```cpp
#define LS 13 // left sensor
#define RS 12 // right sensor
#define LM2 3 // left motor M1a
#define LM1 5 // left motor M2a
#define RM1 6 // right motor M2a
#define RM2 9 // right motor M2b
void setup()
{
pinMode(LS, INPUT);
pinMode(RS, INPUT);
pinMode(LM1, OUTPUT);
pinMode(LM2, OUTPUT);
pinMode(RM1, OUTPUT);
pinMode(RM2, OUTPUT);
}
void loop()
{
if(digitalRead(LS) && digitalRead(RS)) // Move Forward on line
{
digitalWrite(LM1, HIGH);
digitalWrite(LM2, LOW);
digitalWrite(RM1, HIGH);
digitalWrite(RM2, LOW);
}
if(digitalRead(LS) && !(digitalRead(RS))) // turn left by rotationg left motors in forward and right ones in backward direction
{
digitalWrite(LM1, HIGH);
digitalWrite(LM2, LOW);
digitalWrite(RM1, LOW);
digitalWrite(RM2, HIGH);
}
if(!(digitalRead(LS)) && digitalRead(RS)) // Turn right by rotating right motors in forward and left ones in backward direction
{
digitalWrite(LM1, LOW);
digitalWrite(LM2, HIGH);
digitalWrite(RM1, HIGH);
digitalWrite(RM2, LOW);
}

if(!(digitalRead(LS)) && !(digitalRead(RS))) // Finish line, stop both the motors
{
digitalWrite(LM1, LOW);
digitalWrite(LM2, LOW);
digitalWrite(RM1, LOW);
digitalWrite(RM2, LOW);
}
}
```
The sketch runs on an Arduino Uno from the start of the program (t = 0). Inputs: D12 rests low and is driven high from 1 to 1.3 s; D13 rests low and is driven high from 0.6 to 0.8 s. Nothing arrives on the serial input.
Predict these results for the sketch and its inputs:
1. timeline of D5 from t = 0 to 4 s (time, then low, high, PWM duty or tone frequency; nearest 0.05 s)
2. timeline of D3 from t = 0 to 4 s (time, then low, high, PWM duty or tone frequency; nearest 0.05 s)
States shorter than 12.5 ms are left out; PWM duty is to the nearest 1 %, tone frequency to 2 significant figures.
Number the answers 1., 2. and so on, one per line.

1. 0 s low; 0.6 s high; 0.8 s low
2. 0 s low; 1 s high; 1.3 s low
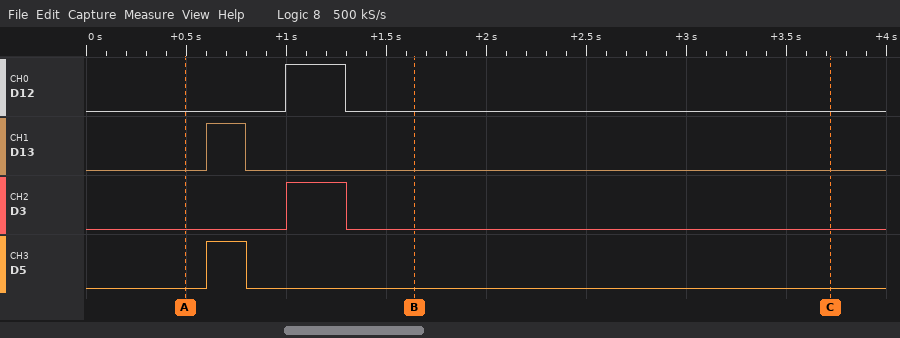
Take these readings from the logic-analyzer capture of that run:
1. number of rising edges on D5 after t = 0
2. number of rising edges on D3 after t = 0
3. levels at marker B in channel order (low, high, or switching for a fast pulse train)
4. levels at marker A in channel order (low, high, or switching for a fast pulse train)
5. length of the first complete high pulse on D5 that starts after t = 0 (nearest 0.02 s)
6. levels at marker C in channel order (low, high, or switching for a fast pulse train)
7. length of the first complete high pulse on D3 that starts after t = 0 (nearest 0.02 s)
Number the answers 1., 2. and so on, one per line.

1. 1
2. 1
3. D12 low, D13 low, D3 low, D5 low
4. D12 low, D13 low, D3 low, D5 low
5. 0.20 s
6. D12 low, D13 low, D3 low, D5 low
7. 0.30 s
